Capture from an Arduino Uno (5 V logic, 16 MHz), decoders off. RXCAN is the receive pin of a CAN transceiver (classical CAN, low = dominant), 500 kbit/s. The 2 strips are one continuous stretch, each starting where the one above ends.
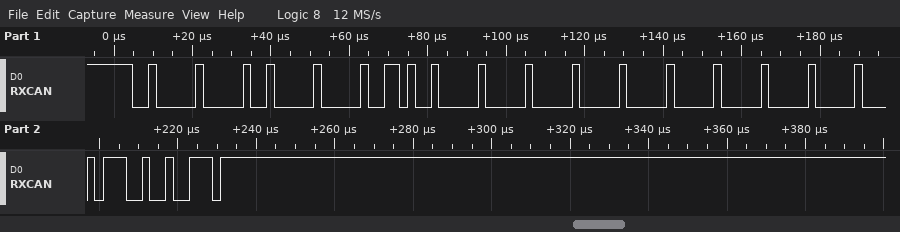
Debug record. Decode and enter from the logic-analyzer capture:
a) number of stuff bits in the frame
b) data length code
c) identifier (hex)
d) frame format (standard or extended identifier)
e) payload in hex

13
8
0x200
standard
00 69 00 00 00 00 00 00
